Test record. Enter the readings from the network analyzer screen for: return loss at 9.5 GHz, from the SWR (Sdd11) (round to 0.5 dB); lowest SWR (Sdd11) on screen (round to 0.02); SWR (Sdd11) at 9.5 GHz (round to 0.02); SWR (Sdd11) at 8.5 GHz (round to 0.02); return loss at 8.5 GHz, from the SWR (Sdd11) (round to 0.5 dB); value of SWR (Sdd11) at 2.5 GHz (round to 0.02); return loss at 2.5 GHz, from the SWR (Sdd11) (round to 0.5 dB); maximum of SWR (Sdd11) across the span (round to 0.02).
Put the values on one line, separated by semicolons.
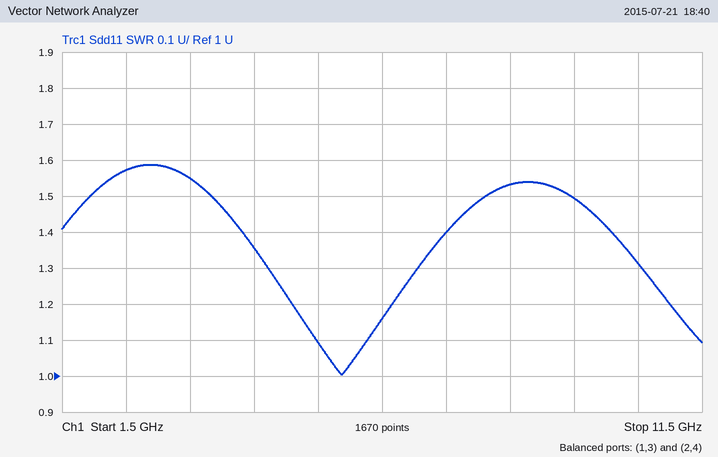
14.0 dB; 1.00; 1.50; 1.54; 13.5 dB; 1.58; 13.0 dB; 1.58
